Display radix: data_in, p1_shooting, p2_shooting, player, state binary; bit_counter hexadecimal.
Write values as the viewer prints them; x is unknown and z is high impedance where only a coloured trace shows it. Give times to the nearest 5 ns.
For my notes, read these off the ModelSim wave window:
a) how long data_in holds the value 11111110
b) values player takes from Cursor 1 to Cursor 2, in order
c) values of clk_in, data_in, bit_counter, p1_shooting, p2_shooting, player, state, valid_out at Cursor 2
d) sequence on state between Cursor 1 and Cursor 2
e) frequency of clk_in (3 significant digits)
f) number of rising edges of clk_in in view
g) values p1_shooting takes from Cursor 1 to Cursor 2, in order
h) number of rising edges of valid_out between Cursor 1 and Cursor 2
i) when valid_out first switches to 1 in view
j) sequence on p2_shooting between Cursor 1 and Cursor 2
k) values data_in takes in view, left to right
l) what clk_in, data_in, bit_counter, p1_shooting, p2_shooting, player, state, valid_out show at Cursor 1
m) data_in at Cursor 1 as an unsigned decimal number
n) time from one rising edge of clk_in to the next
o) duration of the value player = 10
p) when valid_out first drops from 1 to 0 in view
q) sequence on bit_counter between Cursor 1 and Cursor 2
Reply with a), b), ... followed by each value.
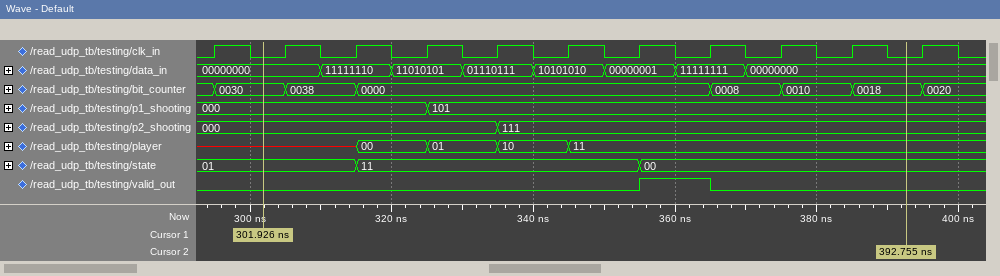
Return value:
a) 10 ns
b) x, 00, 01, 10, 11
c) clk_in=0, data_in=00000000, bit_counter=0018, p1_shooting=101, p2_shooting=111, player=11, state=00, valid_out=0
d) 01, 11, 00
e) 100 MHz
f) 11
g) 000, 101
h) 1
i) 355 ns
j) 000, 111
k) 00000000, 11111110, 11010101, 01110111, 10101010, 00000001, 11111111, 00000000
l) clk_in=0, data_in=00000000, bit_counter=0030, p1_shooting=000, p2_shooting=000, player=x, state=01, valid_out=0
m) 0
n) 10 ns
o) 10 ns
p) 365 ns
q) 0030, 0038, 0000, 0008, 0010, 0018
